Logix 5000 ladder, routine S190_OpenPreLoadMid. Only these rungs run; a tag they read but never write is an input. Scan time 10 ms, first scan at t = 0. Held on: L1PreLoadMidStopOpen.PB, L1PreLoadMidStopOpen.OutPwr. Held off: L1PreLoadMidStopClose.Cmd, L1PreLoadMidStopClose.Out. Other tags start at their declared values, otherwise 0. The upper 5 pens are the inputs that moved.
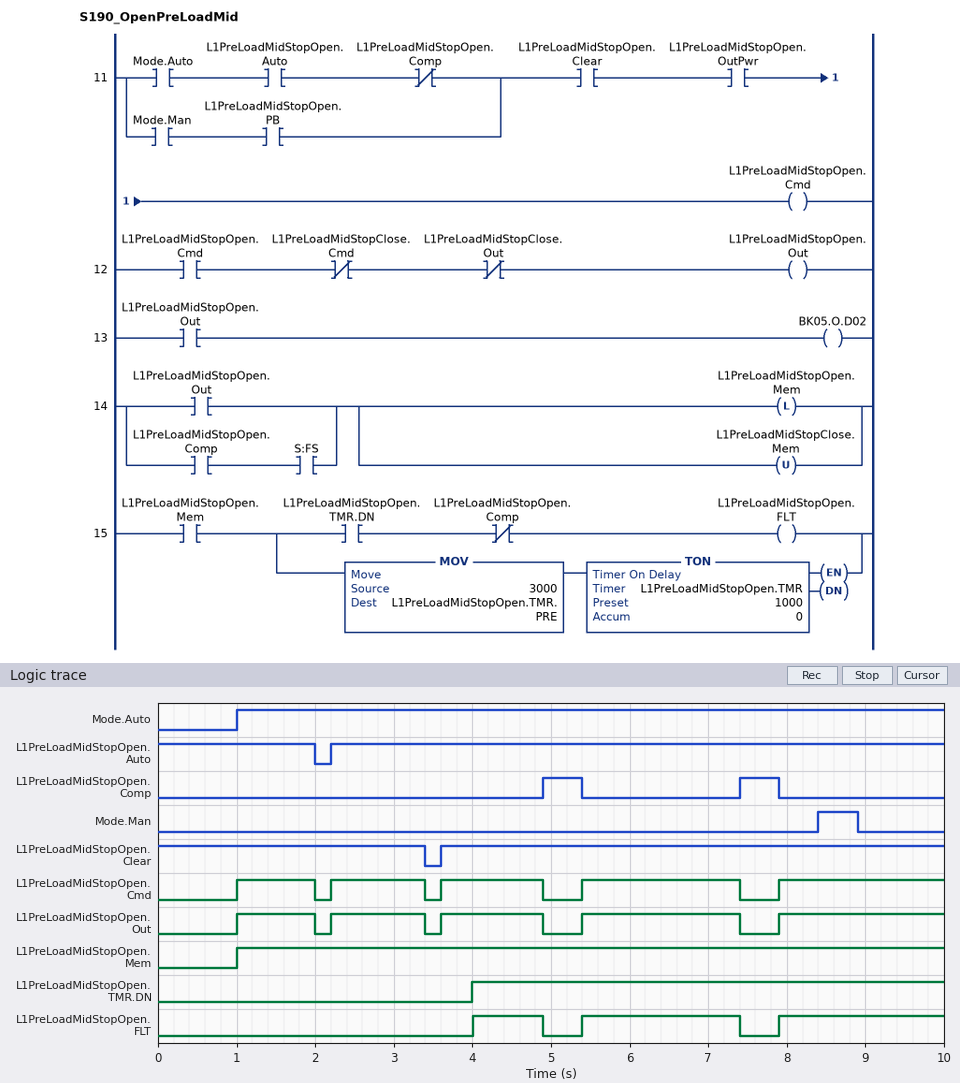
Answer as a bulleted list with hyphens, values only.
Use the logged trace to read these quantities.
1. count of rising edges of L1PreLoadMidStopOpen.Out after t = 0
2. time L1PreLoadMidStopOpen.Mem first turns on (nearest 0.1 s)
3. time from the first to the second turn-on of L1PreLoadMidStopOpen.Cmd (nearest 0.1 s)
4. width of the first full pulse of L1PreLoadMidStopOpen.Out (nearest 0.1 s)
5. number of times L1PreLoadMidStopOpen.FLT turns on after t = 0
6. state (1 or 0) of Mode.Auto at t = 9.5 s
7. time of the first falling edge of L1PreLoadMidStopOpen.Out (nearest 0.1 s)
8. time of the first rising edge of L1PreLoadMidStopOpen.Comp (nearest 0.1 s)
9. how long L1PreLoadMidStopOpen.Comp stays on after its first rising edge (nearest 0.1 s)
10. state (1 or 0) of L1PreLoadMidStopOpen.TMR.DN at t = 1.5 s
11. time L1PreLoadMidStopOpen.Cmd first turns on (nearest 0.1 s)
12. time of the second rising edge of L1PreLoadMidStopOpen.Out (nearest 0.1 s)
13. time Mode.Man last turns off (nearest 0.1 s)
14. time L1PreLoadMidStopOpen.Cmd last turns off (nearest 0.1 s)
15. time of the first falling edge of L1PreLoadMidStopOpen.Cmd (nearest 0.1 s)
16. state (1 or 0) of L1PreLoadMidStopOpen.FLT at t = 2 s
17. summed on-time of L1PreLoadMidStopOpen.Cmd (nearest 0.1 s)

- 5
- 1.0 s
- 1.2 s
- 1.0 s
- 3
- 1
- 2.0 s
- 4.9 s
- 0.5 s
- 0
- 1.0 s
- 2.2 s
- 8.9 s
- 7.4 s
- 2.0 s
- 0
- 7.6 s
